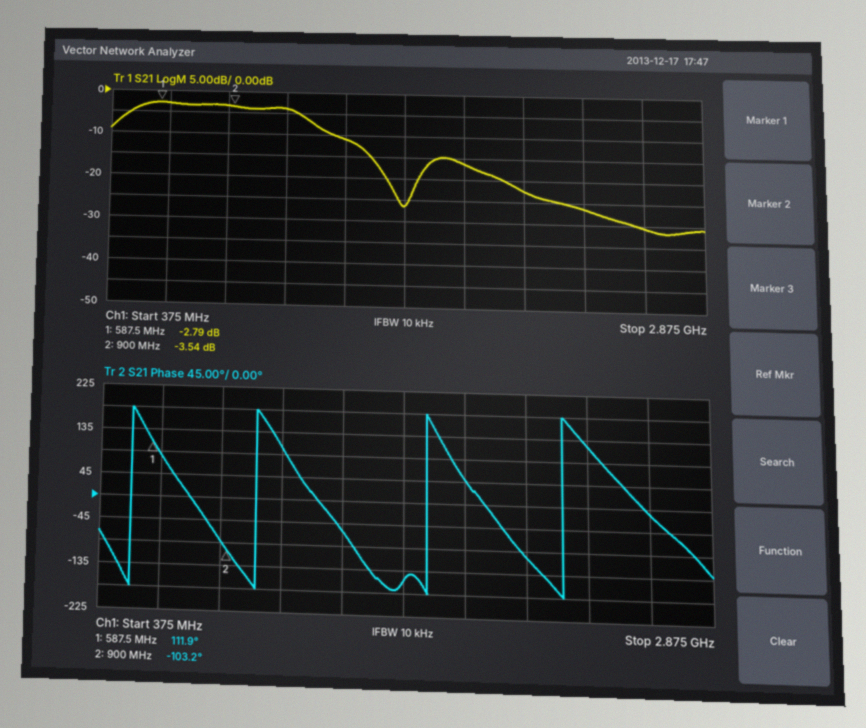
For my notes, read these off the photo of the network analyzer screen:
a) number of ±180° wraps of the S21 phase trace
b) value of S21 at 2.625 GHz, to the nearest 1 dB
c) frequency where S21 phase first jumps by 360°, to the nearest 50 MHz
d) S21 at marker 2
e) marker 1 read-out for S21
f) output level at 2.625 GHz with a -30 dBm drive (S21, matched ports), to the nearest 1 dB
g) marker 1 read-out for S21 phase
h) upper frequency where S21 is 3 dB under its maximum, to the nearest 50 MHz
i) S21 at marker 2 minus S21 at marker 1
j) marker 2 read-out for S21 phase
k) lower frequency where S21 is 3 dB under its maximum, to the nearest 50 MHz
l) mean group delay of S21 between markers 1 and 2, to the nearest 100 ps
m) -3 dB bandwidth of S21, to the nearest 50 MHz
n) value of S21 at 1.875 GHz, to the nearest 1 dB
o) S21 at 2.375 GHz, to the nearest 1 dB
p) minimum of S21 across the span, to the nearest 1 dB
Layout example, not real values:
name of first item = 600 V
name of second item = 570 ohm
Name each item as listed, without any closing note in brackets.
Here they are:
number of ±180° wraps of the S21 phase trace = 4
value of S21 at 2.625 GHz, to the nearest 1 dB = -31 dB
frequency where S21 phase first jumps by 360°, to the nearest 50 MHz = 500 MHz
S21 at marker 2 = -3.54 dB
marker 1 read-out for S21 = -2.79 dB
output level at 2.625 GHz with a -30 dBm drive (S21, matched ports), to the nearest 1 dB = -61 dBm
marker 1 read-out for S21 phase = 111.9°
upper frequency where S21 is 3 dB under its maximum, to the nearest 50 MHz = 1.20 GHz
S21 at marker 2 minus S21 at marker 1 = -0.75 dB
marker 2 read-out for S21 phase = -103.2°
lower frequency where S21 is 3 dB under its maximum, to the nearest 50 MHz = 450 MHz
mean group delay of S21 between markers 1 and 2, to the nearest 100 ps = 1.9 ns
-3 dB bandwidth of S21, to the nearest 50 MHz = 750 MHz
value of S21 at 1.875 GHz, to the nearest 1 dB = -16 dB
S21 at 2.375 GHz, to the nearest 1 dB = -26 dB
minimum of S21 across the span, to the nearest 1 dB = -32 dB
